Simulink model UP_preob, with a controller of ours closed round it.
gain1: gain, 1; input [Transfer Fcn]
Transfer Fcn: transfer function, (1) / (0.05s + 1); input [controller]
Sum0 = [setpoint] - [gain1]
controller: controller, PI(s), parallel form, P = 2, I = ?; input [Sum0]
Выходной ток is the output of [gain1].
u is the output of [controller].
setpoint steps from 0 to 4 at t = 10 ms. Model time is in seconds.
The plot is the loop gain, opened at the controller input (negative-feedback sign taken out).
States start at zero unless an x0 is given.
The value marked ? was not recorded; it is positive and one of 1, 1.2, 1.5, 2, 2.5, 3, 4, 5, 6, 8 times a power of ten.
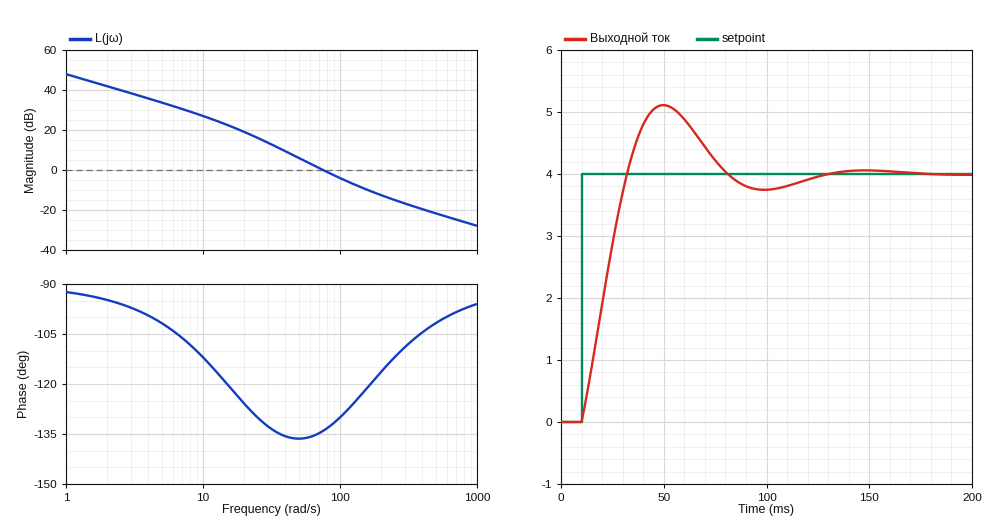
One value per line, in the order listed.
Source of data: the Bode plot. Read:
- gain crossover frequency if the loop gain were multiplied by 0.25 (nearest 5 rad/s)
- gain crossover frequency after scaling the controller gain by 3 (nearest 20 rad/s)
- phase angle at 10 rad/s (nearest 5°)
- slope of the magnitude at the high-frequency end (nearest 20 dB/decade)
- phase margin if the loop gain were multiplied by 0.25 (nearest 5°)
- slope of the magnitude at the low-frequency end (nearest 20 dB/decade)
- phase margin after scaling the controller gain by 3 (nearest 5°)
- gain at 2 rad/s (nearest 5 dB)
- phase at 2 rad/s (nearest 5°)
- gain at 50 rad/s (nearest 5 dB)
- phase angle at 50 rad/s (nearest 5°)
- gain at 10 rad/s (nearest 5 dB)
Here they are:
35 rad/s
160 rad/s
-110°
-20 dB/decade
45°
-20 dB/decade
60°
40 dB
-95°
5 dB
-135°
25 dB
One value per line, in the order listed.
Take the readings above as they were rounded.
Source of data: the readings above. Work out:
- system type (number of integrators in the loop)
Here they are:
1
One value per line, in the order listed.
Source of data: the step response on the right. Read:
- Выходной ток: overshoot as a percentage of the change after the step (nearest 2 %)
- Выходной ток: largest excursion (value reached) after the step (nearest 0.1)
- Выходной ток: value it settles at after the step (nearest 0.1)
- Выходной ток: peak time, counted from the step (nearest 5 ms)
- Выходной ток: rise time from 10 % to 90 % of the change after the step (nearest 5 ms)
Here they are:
28 %
5.1
4.0
40 ms
15 ms
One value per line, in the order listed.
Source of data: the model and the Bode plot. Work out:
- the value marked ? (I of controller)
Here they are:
250
